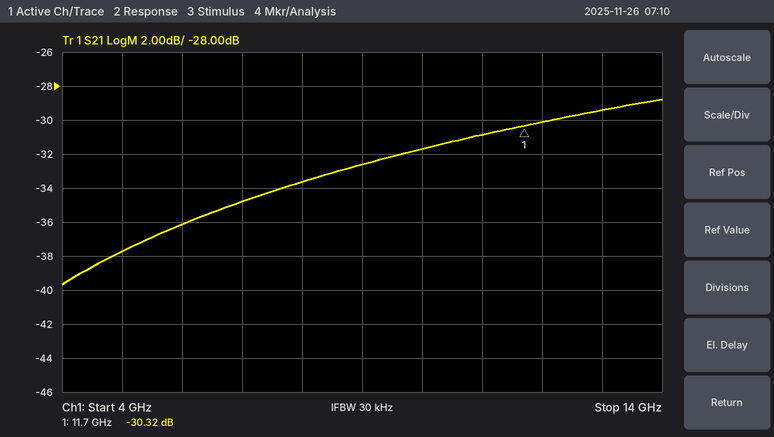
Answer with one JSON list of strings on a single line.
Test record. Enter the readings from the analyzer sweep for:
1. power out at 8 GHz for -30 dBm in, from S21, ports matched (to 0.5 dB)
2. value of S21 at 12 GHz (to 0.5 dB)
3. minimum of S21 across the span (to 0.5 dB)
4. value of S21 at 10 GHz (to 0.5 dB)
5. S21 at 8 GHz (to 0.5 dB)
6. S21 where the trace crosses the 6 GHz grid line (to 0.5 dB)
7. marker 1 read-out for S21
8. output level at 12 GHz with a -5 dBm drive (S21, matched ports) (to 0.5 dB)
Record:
["-63.5 dBm", "-30.0 dB", "-39.5 dB", "-31.5 dB", "-33.5 dB", "-36.0 dB", "-30.32 dB", "-35.0 dBm"]
